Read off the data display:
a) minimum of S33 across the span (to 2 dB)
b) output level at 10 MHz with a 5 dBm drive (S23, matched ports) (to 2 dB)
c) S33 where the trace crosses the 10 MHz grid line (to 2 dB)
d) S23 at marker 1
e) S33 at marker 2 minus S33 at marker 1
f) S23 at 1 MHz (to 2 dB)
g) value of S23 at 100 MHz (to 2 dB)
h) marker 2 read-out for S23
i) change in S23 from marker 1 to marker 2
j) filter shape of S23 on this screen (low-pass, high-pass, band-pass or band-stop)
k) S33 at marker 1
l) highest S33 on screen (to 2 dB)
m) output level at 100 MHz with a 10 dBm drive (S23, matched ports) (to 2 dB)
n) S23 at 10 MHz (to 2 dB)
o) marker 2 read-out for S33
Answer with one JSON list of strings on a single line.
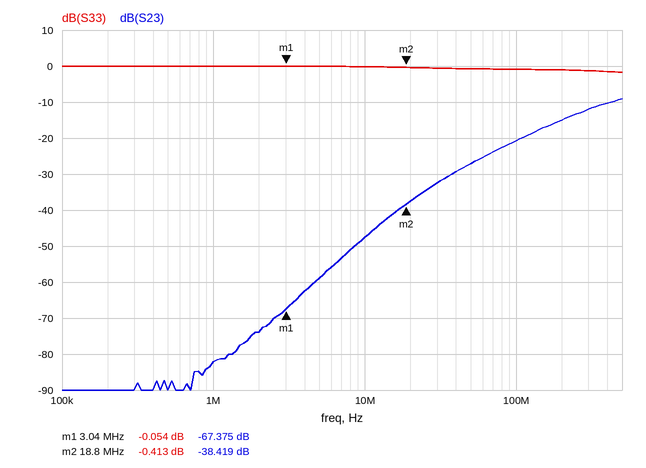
["-2 dB", "-42 dBm", "0 dB", "-67.375 dB", "-0.359 dB", "-82 dB", "-20 dB", "-38.419 dB", "28.956 dB", "high-pass", "-0.054 dB", "0 dB", "-10 dBm", "-48 dB", "-0.413 dB"]
